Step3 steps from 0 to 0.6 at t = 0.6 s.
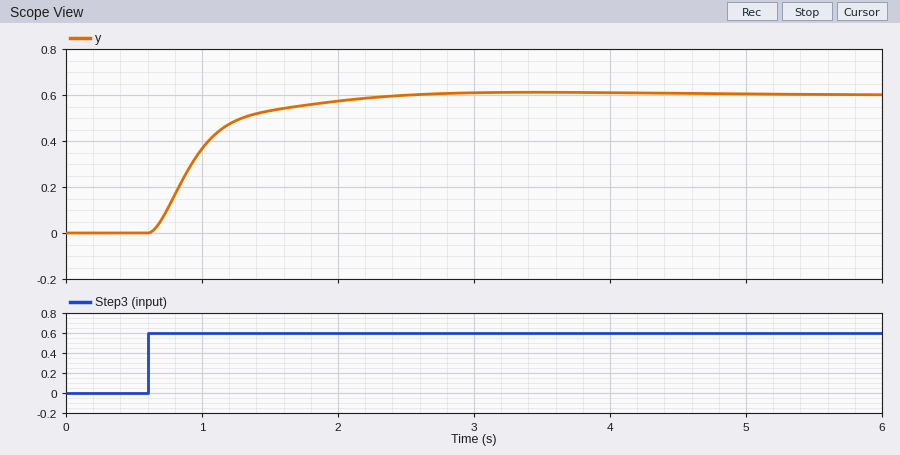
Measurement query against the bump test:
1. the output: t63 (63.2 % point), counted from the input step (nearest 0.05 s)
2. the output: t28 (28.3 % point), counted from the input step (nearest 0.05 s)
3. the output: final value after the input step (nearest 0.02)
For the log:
0.40 s
0.20 s
0.60
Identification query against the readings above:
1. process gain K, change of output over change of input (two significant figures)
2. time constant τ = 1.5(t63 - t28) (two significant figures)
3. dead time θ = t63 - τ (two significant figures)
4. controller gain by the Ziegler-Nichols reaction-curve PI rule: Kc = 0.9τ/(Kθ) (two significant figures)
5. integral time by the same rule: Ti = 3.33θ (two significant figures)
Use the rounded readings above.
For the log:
1.0
0.30 s
0.10 s
2.7
0.33 s
